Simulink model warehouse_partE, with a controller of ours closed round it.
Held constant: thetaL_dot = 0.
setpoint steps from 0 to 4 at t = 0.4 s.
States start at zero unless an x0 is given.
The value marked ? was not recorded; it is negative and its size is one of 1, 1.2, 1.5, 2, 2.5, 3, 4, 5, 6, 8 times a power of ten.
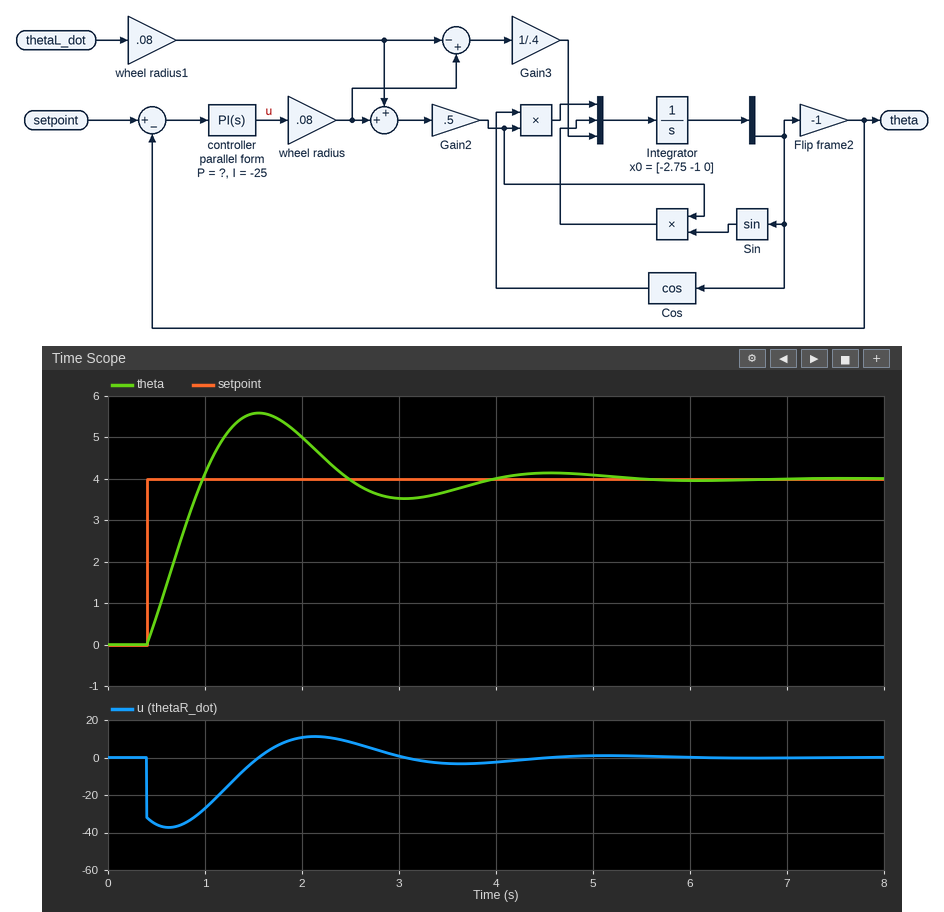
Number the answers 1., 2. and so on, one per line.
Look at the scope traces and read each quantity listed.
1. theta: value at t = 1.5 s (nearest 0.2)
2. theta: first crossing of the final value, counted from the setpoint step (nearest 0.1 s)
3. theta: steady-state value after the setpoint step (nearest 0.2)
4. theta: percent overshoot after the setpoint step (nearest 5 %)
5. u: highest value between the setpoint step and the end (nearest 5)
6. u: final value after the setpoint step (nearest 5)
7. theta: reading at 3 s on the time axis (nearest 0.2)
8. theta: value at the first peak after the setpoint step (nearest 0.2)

1. 5.6
2. 0.6 s
3. 4.0
4. 40 %
5. 10
6. 0
7. 3.6
8. 5.6
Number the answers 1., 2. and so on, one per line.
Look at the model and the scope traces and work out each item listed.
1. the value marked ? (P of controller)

1. -8
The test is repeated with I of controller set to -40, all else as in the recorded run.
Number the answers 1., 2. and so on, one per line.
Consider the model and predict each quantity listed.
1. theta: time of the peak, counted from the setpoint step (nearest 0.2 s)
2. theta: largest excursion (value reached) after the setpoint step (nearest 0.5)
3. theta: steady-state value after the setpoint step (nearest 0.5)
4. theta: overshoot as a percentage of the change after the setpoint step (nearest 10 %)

1. 1.0 s
2. 6.0
3. 4.0
4. 50 %
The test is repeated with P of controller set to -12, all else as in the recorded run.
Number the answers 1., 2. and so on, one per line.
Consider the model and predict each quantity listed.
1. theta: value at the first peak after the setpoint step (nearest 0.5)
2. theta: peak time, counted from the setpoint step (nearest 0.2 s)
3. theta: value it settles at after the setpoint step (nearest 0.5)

1. 5.0
2. 1.0 s
3. 4.0
